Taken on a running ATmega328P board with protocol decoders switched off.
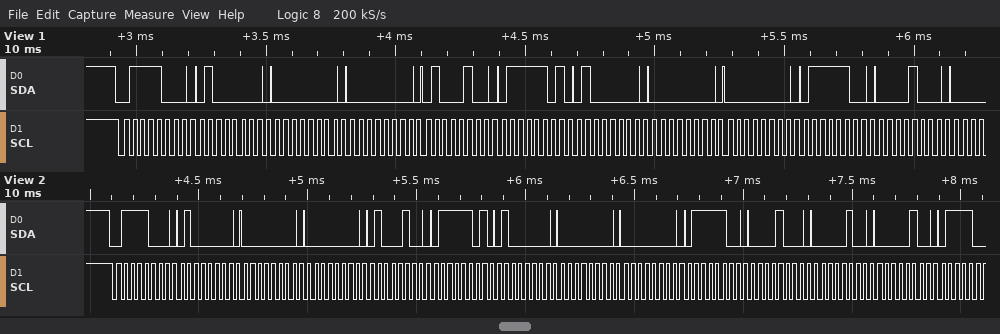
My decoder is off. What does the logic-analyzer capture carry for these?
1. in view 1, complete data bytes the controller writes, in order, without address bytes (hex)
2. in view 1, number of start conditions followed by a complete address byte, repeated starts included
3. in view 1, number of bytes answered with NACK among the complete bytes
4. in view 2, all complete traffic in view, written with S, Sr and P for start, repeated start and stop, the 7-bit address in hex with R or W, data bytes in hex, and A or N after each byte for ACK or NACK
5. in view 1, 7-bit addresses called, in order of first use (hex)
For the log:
40 00 00 44 7D 40 00 00 7C 08
1
0
S 3CW A 40 A 00 A 00 A 44 A 7D A 40 A 00 A 00 A 7C A 08 A 04 A 04 A
0x3C
